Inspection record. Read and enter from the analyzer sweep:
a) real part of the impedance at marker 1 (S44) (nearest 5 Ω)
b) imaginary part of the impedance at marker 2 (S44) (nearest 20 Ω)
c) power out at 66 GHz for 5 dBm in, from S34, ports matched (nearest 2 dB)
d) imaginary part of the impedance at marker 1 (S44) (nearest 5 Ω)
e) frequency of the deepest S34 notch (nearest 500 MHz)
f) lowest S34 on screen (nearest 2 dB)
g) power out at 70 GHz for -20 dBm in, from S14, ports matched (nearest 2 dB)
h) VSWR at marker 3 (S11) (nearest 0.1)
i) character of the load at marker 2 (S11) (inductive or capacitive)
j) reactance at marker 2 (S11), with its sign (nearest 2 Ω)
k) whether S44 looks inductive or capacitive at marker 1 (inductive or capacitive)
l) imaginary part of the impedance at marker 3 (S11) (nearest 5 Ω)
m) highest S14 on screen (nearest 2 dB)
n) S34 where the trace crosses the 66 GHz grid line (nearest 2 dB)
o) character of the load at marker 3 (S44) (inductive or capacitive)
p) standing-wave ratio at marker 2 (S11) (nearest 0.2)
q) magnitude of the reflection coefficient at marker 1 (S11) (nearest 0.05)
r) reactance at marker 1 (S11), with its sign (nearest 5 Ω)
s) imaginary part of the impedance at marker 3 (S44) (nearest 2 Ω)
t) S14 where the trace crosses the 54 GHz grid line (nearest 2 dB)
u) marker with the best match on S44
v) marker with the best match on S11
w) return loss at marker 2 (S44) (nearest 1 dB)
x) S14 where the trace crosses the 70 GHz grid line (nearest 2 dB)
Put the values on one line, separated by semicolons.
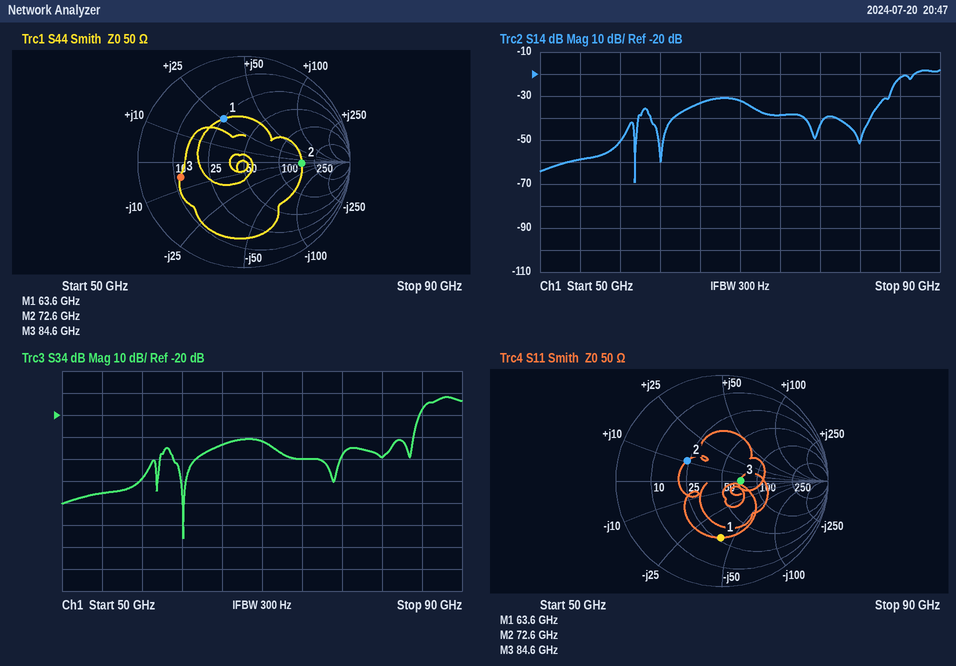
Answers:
25 Ω; 0 Ω; -28 dBm; +25 Ω; 62.0 GHz; -76 dB; -52 dBm; 1.4; inductive; +10 Ω; inductive; 0 Ω; -18 dB; -34 dB; capacitive; 2.2; 0.55; -40 Ω; -6 Ω; -58 dB; marker 1; marker 3; 5 dB; -32 dB
